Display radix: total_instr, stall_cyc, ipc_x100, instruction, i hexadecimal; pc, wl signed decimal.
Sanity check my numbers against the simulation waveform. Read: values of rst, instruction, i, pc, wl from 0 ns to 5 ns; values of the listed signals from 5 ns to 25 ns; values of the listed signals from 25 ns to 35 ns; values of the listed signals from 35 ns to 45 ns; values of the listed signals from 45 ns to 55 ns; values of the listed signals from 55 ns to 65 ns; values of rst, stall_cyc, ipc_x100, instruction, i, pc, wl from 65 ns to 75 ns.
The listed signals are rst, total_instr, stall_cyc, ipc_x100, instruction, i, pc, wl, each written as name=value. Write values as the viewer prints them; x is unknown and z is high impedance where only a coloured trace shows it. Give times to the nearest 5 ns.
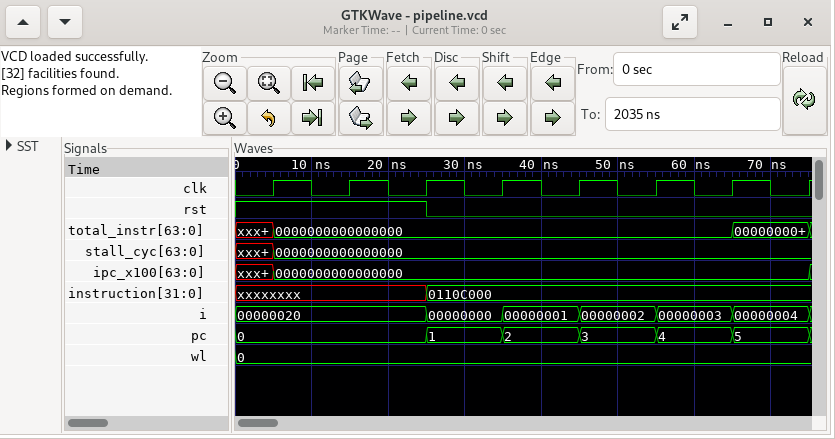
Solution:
rst=1, instruction=xxxxxxxx, i=00000020, pc=0, wl=0
rst=1, total_instr=0000000000000000, stall_cyc=0000000000000000, ipc_x100=0000000000000000, instruction=xxxxxxxx, i=00000020, pc=0, wl=0
rst=0, total_instr=0000000000000000, stall_cyc=0000000000000000, ipc_x100=0000000000000000, instruction=0110C000, i=00000000, pc=1, wl=0
rst=0, total_instr=0000000000000000, stall_cyc=0000000000000000, ipc_x100=0000000000000000, instruction=0110C000, i=00000001, pc=2, wl=0
rst=0, total_instr=0000000000000000, stall_cyc=0000000000000000, ipc_x100=0000000000000000, instruction=0110C000, i=00000002, pc=3, wl=0
rst=0, total_instr=0000000000000000, stall_cyc=0000000000000000, ipc_x100=0000000000000000, instruction=0110C000, i=00000003, pc=4, wl=0
rst=0, stall_cyc=0000000000000000, ipc_x100=0000000000000000, instruction=0110C000, i=00000004, pc=5, wl=0
